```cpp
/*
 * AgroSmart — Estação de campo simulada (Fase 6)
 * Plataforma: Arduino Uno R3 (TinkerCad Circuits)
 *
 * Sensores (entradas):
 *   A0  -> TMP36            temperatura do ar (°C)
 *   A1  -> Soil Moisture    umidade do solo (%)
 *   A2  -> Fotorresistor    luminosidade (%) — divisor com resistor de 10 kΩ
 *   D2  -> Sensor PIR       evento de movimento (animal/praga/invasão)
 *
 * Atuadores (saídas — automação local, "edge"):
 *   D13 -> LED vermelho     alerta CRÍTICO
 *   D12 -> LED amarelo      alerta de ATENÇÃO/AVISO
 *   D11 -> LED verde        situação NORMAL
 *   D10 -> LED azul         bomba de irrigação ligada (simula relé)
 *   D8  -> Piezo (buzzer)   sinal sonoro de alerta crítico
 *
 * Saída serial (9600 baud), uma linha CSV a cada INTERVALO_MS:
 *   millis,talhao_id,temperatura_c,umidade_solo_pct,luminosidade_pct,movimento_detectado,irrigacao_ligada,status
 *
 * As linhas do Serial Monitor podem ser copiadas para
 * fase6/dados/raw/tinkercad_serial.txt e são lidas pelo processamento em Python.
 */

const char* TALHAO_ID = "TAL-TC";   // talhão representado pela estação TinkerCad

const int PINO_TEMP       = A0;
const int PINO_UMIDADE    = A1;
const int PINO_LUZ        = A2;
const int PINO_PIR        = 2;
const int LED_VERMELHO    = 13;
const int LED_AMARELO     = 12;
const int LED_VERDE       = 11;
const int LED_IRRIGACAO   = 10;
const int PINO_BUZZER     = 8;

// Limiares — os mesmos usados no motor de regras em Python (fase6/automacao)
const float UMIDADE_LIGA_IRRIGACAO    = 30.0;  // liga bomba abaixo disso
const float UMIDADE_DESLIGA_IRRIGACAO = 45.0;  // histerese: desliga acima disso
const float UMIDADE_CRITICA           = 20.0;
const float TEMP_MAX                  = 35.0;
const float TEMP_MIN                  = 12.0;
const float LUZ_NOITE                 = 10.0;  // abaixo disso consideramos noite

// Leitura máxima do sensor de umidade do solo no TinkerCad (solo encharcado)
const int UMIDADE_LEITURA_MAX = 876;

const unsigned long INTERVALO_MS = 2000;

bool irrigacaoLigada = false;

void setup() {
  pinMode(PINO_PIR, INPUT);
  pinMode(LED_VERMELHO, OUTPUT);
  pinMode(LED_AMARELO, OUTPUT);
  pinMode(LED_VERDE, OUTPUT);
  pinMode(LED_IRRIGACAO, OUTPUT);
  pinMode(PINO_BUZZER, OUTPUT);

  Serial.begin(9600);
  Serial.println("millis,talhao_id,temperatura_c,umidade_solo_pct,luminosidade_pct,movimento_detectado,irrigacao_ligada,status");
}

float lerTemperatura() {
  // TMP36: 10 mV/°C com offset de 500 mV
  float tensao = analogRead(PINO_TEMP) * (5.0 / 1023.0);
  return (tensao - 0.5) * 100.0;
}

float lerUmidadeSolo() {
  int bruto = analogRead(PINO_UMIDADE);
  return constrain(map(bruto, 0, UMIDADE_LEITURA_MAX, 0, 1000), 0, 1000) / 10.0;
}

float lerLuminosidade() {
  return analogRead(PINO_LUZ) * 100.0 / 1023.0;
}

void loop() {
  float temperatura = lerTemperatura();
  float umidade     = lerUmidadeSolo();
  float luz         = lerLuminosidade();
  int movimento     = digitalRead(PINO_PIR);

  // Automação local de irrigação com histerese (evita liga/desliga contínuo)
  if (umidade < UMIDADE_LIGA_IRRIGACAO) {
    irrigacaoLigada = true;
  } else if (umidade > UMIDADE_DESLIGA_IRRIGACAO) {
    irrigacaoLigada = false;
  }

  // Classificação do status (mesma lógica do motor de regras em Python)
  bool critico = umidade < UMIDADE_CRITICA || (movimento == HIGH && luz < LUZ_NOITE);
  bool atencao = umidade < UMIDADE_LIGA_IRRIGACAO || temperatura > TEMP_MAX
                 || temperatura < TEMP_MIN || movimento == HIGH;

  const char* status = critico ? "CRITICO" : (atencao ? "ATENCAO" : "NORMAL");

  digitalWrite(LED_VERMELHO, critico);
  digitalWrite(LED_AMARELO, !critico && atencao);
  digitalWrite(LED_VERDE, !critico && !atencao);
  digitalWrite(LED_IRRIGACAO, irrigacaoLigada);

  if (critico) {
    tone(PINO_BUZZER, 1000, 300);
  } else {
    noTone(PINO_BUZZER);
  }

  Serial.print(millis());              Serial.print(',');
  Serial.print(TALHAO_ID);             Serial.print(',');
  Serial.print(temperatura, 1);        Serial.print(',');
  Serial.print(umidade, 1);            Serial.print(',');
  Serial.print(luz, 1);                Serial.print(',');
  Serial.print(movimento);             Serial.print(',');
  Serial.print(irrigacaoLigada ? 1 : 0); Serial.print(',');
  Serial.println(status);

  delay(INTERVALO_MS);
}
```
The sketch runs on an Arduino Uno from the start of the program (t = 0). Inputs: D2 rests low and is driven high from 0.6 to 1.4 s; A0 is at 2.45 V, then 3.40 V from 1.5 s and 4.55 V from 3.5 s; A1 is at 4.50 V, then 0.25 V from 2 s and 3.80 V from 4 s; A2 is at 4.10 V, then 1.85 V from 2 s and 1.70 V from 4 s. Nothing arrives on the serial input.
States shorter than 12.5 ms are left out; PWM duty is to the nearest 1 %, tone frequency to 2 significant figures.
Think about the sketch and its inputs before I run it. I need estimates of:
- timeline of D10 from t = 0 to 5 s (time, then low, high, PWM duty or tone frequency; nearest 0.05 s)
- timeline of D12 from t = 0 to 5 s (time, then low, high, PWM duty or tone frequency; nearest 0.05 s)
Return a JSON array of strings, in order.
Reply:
["0 s low; 2.1 s high; 4.1 s low", "0 s low; 0.05 s high; 2.1 s low; 4.1 s high"]
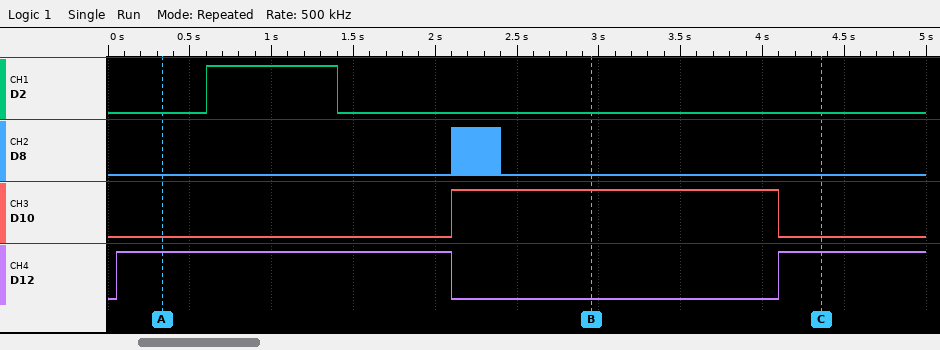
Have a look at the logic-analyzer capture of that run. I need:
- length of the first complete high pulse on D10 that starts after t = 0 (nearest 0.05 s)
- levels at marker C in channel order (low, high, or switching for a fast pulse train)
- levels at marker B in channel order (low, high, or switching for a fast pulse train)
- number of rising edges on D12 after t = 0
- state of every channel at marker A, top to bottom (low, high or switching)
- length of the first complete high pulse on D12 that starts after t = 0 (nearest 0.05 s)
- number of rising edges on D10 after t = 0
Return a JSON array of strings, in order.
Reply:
["2.00 s", "D2 low, D8 low, D10 low, D12 high", "D2 low, D8 low, D10 high, D12 low", "2", "D2 low, D8 low, D10 low, D12 high", "2.05 s", "1"]
